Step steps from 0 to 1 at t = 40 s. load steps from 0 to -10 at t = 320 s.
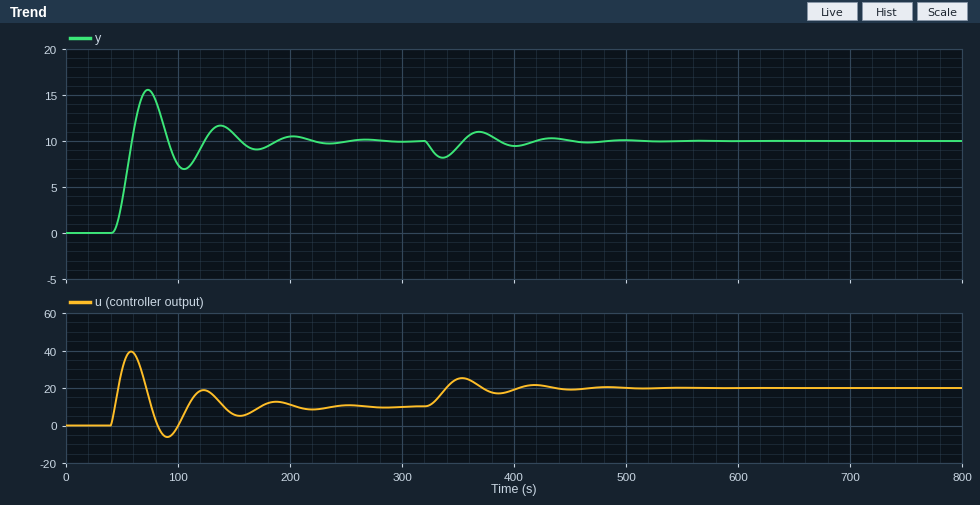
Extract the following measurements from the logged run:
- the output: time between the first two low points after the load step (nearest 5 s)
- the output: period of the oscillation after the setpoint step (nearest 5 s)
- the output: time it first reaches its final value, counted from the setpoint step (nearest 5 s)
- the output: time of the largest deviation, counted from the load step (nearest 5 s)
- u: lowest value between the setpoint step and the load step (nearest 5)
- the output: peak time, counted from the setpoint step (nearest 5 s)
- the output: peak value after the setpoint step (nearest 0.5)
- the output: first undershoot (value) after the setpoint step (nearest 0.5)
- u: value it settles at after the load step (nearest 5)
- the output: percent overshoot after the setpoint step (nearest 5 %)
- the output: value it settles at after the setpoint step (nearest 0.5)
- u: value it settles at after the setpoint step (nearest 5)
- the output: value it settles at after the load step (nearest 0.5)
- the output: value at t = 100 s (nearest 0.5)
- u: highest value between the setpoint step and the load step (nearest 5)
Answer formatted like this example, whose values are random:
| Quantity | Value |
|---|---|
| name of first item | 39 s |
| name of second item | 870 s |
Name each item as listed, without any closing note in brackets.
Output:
| Quantity | Value |
|---|---|
| the output: time between the first two low points after the load step | 65 s |
| the output: period of the oscillation after the setpoint step | 65 s |
| the output: time it first reaches its final value, counted from the setpoint step | 20 s |
| the output: time of the largest deviation, counted from the load step | 15 s |
| u: lowest value between the setpoint step and the load step | -5 |
| the output: peak time, counted from the setpoint step | 35 s |
| the output: peak value after the setpoint step | 15.5 |
| the output: first undershoot (value) after the setpoint step | 7.0 |
| u: value it settles at after the load step | 20 |
| the output: percent overshoot after the setpoint step | 55 % |
| the output: value it settles at after the setpoint step | 10.0 |
| u: value it settles at after the setpoint step | 10 |
| the output: value it settles at after the load step | 10.0 |
| the output: value at t = 100 s | 7.5 |
| u: highest value between the setpoint step and the load step | 40 |
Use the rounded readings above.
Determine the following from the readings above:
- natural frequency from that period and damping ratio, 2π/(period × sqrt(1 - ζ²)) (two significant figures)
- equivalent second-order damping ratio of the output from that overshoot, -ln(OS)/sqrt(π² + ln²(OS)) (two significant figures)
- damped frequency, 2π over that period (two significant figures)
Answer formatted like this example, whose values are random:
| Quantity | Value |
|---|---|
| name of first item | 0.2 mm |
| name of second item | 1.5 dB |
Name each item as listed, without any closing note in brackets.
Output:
| Quantity | Value |
|---|---|
| natural frequency from that period and damping ratio, 2π/(period × sqrt(1 - ζ²)) | 0.098 rad/s |
| equivalent second-order damping ratio of the output from that overshoot, -ln(OS)/sqrt(π² + ln²(OS)) | 0.19 |
| damped frequency, 2π over that period | 0.097 rad/s |
